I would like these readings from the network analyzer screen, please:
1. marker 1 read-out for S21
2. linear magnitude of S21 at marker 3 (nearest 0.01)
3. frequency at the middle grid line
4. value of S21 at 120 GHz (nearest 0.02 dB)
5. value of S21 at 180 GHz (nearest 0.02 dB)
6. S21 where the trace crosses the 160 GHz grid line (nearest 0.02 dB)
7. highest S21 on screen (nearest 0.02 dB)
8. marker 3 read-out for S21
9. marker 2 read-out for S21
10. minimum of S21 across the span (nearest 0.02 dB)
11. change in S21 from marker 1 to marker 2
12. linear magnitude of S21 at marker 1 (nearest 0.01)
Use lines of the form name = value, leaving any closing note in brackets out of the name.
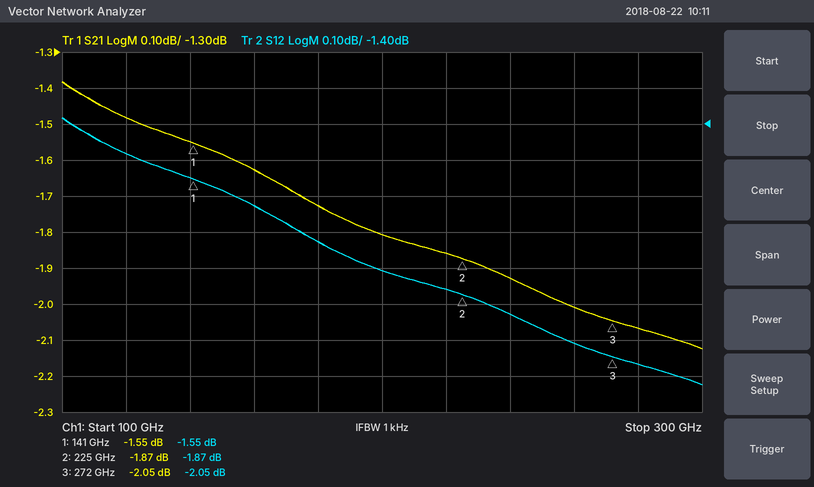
marker 1 read-out for S21 = -1.55 dB
linear magnitude of S21 at marker 3 = 0.79
frequency at the middle grid line = 200 GHz
value of S21 at 120 GHz = -1.48 dB
value of S21 at 180 GHz = -1.72 dB
S21 where the trace crosses the 160 GHz grid line = -1.62 dB
highest S21 on screen = -1.38 dB
marker 3 read-out for S21 = -2.05 dB
marker 2 read-out for S21 = -1.87 dB
minimum of S21 across the span = -2.12 dB
change in S21 from marker 1 to marker 2 = -0.32 dB
linear magnitude of S21 at marker 1 = 0.84
